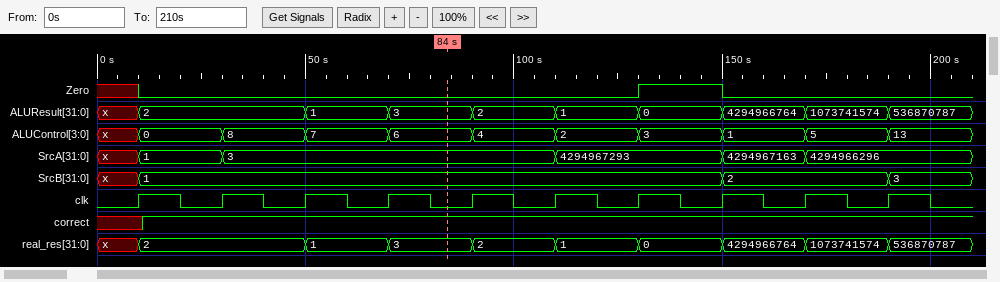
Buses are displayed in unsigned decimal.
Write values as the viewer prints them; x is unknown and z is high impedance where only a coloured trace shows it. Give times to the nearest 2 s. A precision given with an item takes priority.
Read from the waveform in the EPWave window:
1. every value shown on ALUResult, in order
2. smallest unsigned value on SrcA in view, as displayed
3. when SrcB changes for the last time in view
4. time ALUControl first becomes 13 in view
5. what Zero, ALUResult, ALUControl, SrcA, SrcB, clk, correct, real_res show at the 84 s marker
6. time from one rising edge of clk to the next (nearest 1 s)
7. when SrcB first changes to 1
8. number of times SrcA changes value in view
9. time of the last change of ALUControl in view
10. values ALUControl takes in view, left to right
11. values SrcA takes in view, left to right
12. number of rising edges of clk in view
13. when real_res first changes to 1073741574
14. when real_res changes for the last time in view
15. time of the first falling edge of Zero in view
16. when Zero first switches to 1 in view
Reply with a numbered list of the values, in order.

1. x, 2, 1, 3, 2, 1, 0, 4294966764, 1073741574, 536870787
2. 1
3. 190 s
4. 190 s
5. Zero=0, ALUResult=3, ALUControl=6, SrcA=3, SrcB=1, clk=0, correct=1, real_res=3
6. 20 s
7. 10 s
8. 5
9. 190 s
10. x, 0, 8, 7, 6, 4, 2, 3, 1, 5, 13
11. x, 1, 3, 4294967293, 4294967163, 4294966296
12. 10
13. 170 s
14. 190 s
15. 150 s
16. 130 s
